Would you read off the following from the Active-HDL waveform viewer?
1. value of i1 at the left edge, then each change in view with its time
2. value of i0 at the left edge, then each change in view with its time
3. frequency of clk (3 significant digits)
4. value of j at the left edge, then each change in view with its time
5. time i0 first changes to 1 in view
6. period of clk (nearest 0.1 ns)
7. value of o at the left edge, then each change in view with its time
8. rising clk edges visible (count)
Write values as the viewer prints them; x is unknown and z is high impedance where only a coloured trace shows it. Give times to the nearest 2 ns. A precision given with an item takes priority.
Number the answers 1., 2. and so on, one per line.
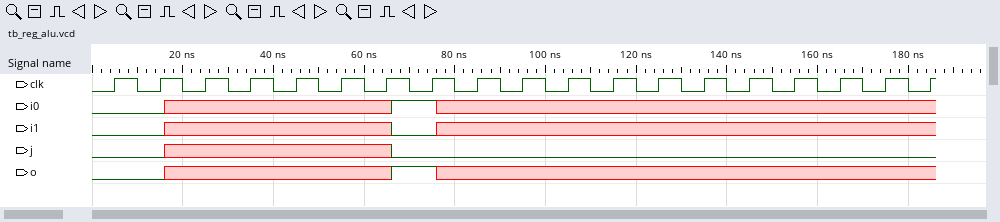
1. 0, x at 16 ns, 0 at 66 ns, x at 76 ns
2. 0, x at 16 ns, 1 at 66 ns, x at 76 ns
3. 100 MHz
4. 0, x at 16 ns, 0 at 66 ns
5. 66 ns
6. 10 ns
7. 0, x at 16 ns, 1 at 66 ns, x at 76 ns
8. 19
